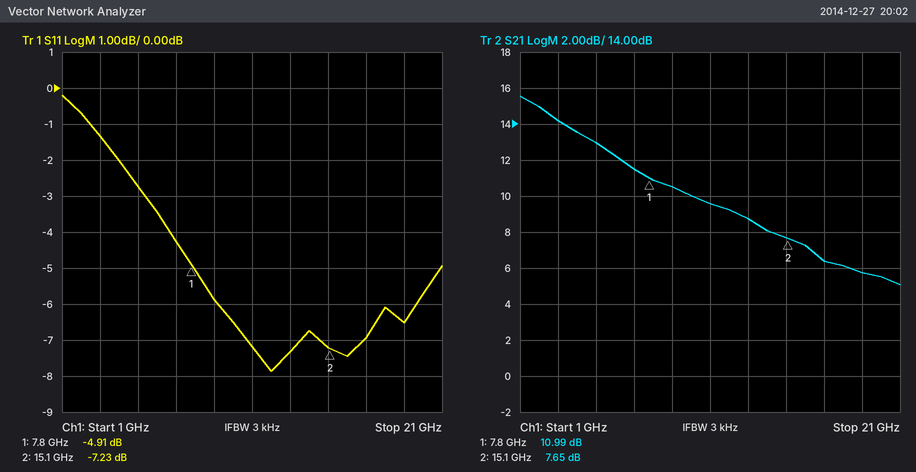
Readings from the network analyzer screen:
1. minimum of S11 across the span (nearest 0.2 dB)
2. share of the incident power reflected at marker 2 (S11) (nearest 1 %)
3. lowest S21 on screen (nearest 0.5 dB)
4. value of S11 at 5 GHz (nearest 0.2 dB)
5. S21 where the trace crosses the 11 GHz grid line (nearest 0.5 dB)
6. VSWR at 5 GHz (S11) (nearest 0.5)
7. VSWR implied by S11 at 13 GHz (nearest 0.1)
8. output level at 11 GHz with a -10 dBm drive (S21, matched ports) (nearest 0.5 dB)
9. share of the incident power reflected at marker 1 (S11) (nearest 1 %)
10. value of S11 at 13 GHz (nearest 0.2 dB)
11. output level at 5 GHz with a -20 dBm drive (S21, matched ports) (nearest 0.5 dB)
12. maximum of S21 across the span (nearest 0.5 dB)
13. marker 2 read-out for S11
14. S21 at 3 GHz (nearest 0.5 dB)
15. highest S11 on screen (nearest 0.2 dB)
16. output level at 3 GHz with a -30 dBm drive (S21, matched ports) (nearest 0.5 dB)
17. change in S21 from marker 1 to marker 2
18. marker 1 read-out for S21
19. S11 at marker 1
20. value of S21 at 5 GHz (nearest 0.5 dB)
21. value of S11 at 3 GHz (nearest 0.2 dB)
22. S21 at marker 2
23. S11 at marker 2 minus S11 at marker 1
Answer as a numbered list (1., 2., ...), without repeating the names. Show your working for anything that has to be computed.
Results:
1. -7.8 dB
2. 10^(-7.23/10) ≈ 19 %
3. 5.0 dB
4. -2.8 dB
5. 9.5 dB
6. |Γ| = 10^(-2.8/20) = 0.7244; VSWR = (1 + 0.7244)/(1 − 0.7244) ≈ 6.26, so 6.5 to the nearest 0.5
7. |Γ| = 10^(-7.4/20) = 0.4266; VSWR = (1 + 0.4266)/(1 − 0.4266) ≈ 2.5
8. -10 dBm + (9.5 dB) = -0.5 dBm
9. 10^(-4.91/10) ≈ 32 %
10. -7.4 dB
11. -20 dBm + (13.0 dB) = -7.0 dBm
12. 15.5 dB
13. -7.23 dB
14. 14.0 dB
15. -0.2 dB
16. -30 dBm + (14.0 dB) = -16.0 dBm
17. 7.65 − (10.99) = -3.34 dB
18. 10.99 dB
19. -4.91 dB
20. 13.0 dB
21. -1.4 dB
22. 7.65 dB
23. -7.23 − (-4.91) = -2.32 dB
